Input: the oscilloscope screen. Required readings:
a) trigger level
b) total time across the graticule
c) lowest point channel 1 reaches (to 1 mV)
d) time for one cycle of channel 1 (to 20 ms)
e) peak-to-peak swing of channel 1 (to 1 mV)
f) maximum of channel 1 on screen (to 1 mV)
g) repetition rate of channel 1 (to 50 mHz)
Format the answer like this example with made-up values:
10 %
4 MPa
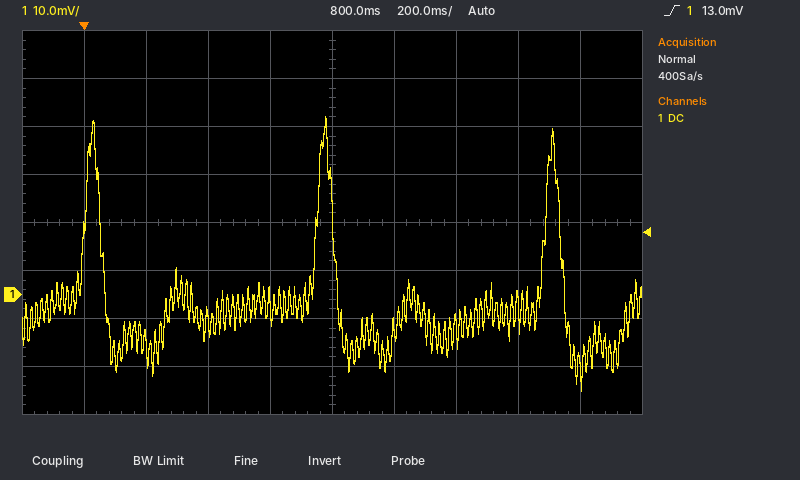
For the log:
13.0 mV
2 s
-20 mV
740 ms
57 mV
37 mV
1.35 Hz
